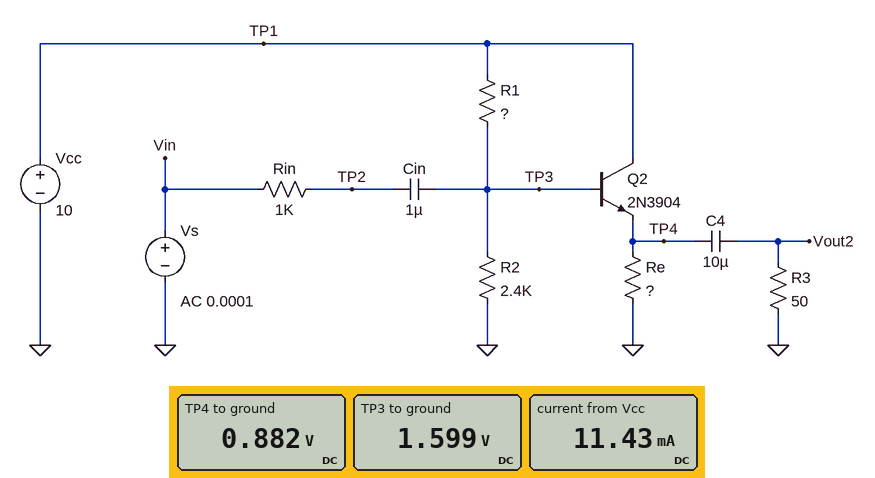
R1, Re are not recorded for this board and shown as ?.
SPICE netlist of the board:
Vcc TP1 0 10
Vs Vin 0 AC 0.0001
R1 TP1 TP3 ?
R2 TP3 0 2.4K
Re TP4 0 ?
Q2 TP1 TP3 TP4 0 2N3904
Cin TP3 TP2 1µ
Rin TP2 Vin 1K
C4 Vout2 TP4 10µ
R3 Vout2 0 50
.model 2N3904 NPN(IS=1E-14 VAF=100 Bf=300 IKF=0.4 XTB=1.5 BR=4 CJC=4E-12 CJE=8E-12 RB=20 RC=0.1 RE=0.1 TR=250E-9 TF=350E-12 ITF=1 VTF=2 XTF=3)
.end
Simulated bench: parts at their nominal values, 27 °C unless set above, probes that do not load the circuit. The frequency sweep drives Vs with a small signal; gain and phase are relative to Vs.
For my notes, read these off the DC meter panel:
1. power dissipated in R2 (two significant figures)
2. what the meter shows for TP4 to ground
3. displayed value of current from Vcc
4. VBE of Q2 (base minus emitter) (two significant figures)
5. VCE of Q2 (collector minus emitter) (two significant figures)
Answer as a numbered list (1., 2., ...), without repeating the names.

1. 1.1 mW
2. 0.882 V
3. 11.43 mA
4. 720 mV
5. 9.1 V
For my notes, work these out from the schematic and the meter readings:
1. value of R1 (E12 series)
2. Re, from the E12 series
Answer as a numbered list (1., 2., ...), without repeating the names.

1. 12 kΩ
2. 82 Ω
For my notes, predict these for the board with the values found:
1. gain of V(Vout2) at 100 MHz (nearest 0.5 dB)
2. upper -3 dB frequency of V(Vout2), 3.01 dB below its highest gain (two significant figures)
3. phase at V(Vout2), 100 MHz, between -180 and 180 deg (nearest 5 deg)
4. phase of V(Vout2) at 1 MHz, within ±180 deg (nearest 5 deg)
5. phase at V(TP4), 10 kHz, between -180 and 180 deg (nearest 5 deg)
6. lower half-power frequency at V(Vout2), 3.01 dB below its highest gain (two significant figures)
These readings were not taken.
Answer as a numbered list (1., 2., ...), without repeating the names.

1. -19.5 dB
2. 18 MHz
3. -70 deg
4. -5 deg
5. 0 deg
6. 310 Hz
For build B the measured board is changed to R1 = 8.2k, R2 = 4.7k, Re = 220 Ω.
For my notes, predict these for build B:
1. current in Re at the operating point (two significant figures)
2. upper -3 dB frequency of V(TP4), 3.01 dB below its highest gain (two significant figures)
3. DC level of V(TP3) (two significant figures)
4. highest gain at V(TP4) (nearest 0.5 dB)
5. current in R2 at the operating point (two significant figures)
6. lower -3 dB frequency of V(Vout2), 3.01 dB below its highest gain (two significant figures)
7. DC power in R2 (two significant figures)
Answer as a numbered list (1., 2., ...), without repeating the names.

1. 13 mA
2. 19 MHz
3. 3.5 V
4. -3.0 dB
5. 750 µA
6. 300 Hz
7. 2.6 mW
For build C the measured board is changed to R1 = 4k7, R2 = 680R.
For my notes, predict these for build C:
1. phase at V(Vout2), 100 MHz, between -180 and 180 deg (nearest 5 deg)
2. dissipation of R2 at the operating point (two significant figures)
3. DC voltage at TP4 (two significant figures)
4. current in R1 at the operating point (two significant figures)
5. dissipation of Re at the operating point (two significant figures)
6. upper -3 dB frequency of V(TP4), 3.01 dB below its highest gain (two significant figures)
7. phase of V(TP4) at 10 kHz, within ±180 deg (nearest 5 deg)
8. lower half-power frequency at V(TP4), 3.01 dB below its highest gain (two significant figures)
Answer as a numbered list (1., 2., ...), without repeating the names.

1. -60 deg
2. 2.3 mW
3. 550 mV
4. 1.9 mA
5. 3.7 mW
6. 30 MHz
7. 0 deg
8. 87 Hz
